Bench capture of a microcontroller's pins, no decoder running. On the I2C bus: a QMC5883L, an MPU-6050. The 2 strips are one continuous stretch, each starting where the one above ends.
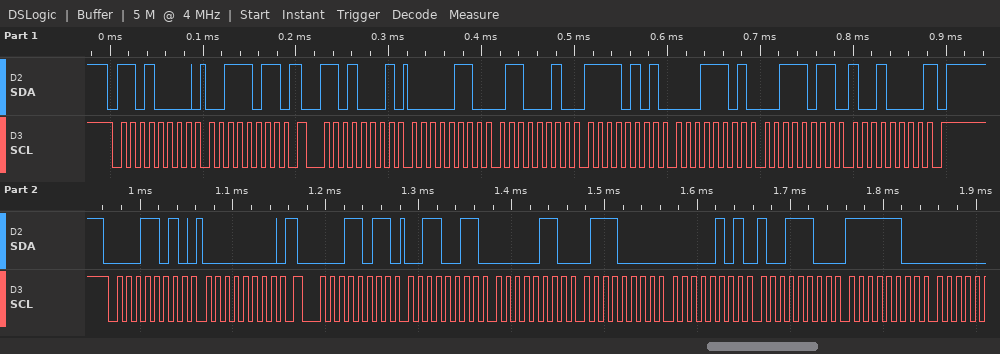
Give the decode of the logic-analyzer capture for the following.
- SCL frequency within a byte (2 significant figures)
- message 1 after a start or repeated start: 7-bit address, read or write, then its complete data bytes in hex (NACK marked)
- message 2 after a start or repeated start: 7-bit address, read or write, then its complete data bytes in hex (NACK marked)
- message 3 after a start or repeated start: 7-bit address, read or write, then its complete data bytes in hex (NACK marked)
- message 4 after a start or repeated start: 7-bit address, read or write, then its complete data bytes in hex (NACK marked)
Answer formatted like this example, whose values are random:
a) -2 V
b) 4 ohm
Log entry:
a) 100 kHz
b) 0x68 write: 3B
c) 0x68 read: 06 62 F5 1D 3B 90 NACK
d) 0x0D write: 00
e) 0x0D read: 33 06 70 05 9C FC
